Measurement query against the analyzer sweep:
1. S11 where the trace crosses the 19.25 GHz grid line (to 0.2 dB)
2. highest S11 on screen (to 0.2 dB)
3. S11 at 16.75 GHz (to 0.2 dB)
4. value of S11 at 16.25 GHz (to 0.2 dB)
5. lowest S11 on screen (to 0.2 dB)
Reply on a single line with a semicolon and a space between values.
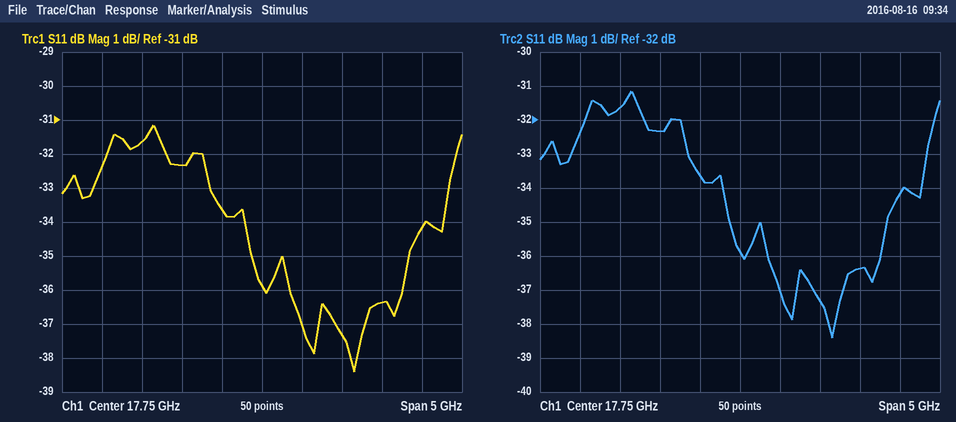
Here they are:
-36.4 dB; -31.2 dB; -32.4 dB; -31.6 dB; -38.4 dB
